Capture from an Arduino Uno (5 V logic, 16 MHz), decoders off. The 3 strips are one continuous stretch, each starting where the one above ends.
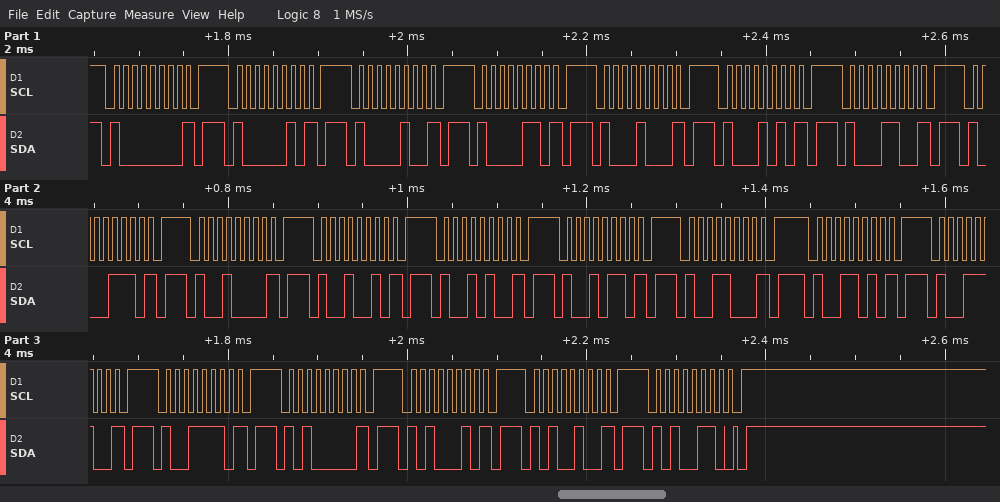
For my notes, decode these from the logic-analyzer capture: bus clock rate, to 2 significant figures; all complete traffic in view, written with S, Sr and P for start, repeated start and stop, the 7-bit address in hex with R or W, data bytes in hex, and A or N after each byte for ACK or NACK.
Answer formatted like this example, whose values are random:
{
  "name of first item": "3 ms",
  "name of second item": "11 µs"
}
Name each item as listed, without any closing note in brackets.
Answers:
{
  "bus clock rate, to 2 significant figures": "100 kHz",
  "all complete traffic in view, written with S, Sr and P for start, repeated start and stop, the 7-bit address in hex with R or W, data bytes in hex, and A or N after each byte for ACK or NACK": "S 40W N P S 41W N P S 42W N P S 43W N P S 44W N P S 45W N P S 46W N P S 47W N P S 48W N P S 49W N P S 4AW N P S 4BW N P S 4CW N P S 4DW N P S 4EW N P S 4FW N P S 50W N P S 51W N P S 52W N P S 53W A P"
}
